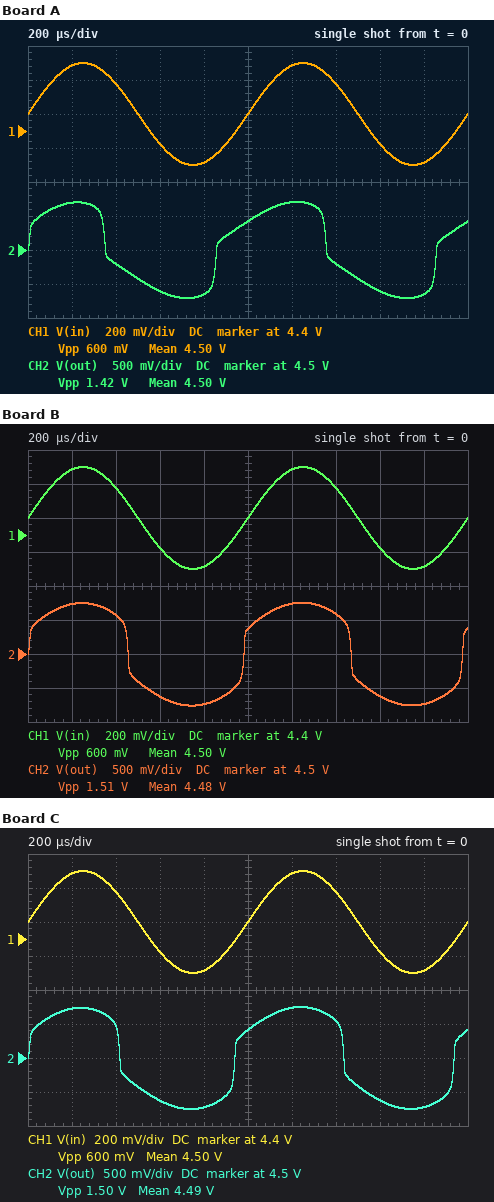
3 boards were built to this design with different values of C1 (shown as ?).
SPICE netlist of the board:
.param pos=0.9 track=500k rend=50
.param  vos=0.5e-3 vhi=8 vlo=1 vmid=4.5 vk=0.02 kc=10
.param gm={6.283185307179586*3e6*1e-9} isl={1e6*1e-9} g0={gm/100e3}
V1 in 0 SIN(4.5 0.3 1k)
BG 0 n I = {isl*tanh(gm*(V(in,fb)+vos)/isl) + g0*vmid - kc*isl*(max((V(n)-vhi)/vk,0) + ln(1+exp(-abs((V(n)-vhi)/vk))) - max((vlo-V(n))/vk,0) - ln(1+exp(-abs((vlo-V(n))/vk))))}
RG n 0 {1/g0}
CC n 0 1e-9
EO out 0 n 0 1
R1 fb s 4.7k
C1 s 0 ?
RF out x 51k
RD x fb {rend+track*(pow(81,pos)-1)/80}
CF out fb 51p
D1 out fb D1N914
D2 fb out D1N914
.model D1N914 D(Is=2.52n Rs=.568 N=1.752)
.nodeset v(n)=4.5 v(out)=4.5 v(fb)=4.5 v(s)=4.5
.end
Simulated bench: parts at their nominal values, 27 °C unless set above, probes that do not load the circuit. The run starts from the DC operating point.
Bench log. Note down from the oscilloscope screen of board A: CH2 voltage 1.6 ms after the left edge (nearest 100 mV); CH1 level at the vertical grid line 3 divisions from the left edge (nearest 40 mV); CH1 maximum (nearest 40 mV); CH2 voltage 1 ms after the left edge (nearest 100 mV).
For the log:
3.9 V
4.32 V
4.80 V
4.9 V
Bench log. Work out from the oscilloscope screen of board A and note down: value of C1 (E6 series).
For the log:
22 nF
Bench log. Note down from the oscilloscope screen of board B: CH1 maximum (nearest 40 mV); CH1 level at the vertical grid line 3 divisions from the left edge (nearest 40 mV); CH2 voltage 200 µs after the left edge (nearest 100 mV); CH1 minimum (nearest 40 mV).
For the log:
4.80 V
4.32 V
5.2 V
4.20 V
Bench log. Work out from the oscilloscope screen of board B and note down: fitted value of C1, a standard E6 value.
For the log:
150 nF
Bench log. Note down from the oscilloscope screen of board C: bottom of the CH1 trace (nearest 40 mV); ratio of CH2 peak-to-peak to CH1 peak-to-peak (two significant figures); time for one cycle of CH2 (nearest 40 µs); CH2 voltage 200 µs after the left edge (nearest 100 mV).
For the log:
4.20 V
2.5
1.00 ms
5.2 V
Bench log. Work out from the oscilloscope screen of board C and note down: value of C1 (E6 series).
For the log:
68 nF
